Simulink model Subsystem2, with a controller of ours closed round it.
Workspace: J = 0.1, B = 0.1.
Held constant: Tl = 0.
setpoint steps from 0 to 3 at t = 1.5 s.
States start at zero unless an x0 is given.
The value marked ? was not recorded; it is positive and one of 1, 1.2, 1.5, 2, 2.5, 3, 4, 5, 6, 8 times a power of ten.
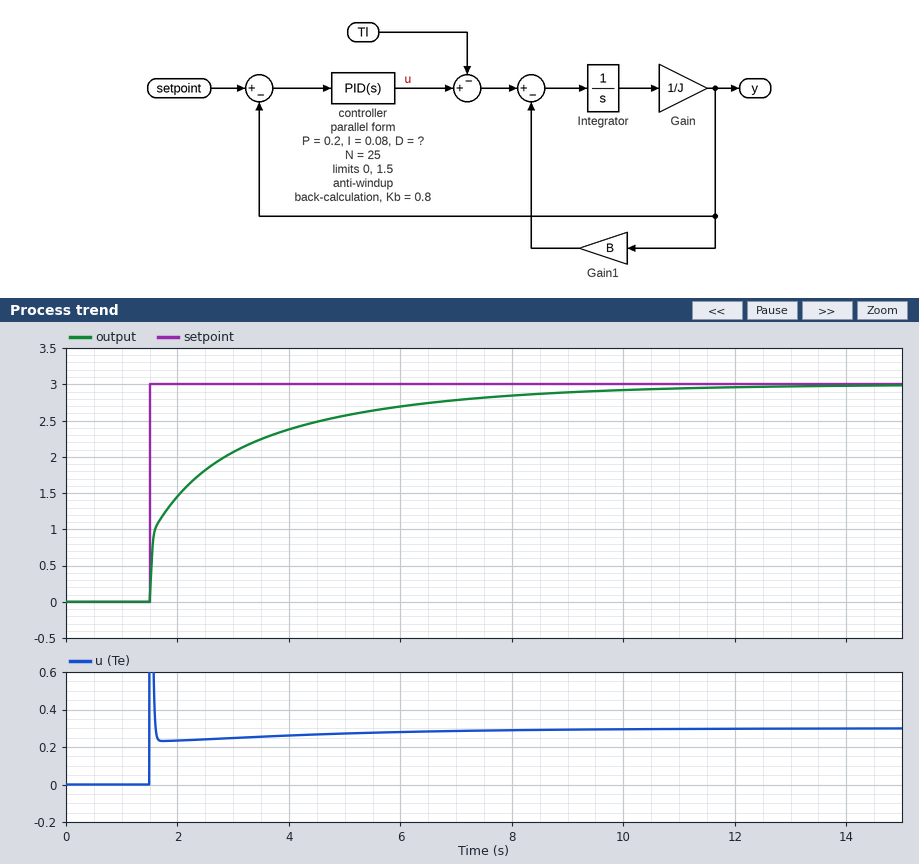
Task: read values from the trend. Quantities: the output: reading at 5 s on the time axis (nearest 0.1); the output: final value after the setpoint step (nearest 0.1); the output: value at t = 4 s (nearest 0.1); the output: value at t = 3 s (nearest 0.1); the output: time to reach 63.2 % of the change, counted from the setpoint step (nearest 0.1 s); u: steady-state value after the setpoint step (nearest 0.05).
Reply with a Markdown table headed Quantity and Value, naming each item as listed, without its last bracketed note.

| Quantity | Value |
|---|---|
| the output: reading at 5 s on the time axis | 2.6 |
| the output: final value after the setpoint step | 3.0 |
| the output: value at t = 4 s | 2.4 |
| the output: value at t = 3 s | 2.1 |
| the output: time to reach 63.2 % of the change, counted from the setpoint step | 1.1 s |
| u: steady-state value after the setpoint step | 0.30 |
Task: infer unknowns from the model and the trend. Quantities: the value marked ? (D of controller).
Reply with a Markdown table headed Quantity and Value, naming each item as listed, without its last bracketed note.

| Quantity | Value |
|---|---|
| the value marked ? | 0.08 |
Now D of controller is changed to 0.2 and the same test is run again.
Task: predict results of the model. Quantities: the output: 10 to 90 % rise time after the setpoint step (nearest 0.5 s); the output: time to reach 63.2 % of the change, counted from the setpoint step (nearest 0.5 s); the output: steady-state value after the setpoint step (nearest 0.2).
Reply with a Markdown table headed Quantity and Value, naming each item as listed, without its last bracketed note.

| Quantity | Value |
|---|---|
| the output: 10 to 90 % rise time after the setpoint step | 6.0 s |
| the output: time to reach 63.2 % of the change, counted from the setpoint step | 2.5 s |
| the output: steady-state value after the setpoint step | 3.0 |
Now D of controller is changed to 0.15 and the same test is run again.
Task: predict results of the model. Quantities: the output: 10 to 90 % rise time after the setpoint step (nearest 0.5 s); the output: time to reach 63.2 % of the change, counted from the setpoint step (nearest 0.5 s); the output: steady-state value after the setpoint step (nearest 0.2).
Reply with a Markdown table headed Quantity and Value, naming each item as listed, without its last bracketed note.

| Quantity | Value |
|---|---|
| the output: 10 to 90 % rise time after the setpoint step | 5.5 s |
| the output: time to reach 63.2 % of the change, counted from the setpoint step | 2.0 s |
| the output: steady-state value after the setpoint step | 3.0 |
